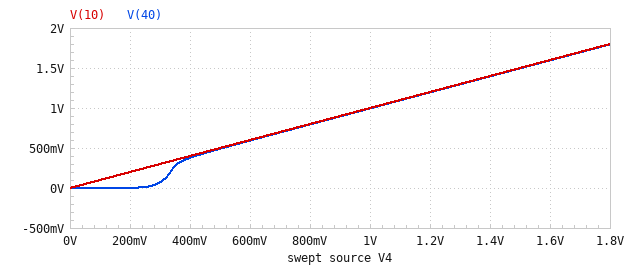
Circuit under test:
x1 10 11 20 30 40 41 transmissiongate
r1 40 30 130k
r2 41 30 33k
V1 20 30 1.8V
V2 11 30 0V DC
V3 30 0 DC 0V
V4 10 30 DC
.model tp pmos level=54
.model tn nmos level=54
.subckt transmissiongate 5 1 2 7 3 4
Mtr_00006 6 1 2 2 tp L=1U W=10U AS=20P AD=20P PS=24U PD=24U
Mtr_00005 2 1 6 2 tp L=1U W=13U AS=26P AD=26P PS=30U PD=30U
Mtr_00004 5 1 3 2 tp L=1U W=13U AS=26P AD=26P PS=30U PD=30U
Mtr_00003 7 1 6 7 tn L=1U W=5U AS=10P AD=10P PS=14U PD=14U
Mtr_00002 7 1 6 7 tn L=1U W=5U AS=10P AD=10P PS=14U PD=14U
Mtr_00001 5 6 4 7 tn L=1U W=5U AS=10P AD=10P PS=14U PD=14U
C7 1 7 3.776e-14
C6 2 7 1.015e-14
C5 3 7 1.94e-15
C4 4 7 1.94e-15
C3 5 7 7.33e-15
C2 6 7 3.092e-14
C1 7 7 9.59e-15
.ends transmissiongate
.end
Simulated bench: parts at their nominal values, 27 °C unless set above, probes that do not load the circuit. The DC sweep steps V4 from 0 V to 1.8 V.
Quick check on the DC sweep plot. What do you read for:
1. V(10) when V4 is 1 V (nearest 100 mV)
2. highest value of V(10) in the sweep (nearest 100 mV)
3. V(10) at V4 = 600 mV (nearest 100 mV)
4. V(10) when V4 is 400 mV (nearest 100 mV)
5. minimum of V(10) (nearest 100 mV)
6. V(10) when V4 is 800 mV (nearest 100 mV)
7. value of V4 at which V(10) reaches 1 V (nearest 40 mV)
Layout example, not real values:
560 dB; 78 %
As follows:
1.0 V; 1.8 V; 600 mV; 400 mV; 0 V; 800 mV; 1.00 V
